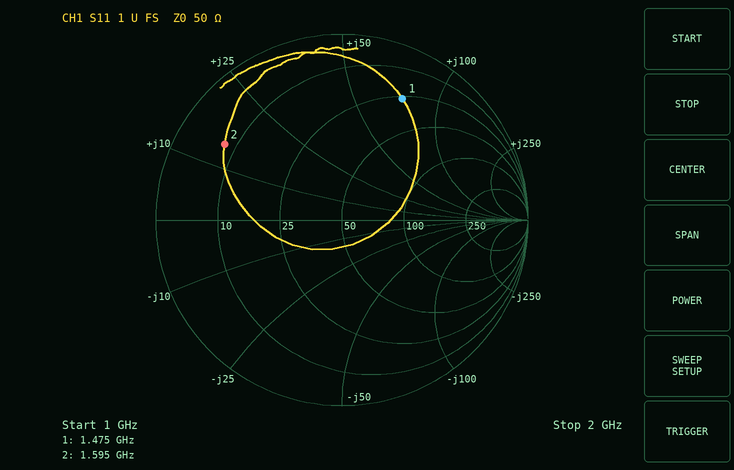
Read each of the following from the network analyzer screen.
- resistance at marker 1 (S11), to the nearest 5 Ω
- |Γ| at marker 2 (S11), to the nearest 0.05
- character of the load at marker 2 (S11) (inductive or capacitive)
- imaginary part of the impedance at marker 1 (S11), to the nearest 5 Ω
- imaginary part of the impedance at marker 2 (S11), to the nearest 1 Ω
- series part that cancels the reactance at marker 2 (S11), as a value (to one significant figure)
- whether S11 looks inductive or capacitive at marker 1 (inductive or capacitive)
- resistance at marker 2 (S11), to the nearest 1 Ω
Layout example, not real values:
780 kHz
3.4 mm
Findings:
25 Ω
0.75
inductive
+75 Ω
+14 Ω
7 pF
inductive
8 Ω
